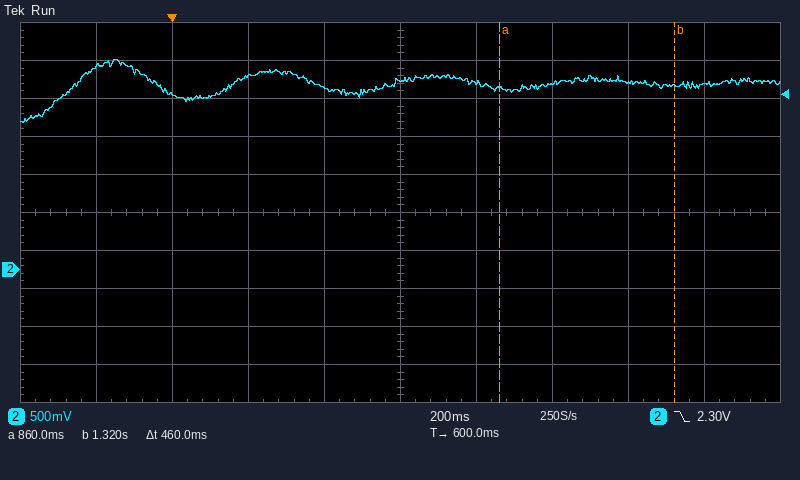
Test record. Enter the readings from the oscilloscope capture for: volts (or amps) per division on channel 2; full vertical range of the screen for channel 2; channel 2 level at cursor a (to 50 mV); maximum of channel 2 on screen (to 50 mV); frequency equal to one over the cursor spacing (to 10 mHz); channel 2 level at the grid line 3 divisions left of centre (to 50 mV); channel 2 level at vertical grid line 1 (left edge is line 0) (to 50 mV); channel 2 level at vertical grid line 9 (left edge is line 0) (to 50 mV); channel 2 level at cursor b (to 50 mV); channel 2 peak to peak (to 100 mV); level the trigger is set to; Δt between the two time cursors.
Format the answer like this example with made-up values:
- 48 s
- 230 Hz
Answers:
- 500 mV
- 5 V
- 2.40 V
- 2.75 V
- 2.17 Hz
- 2.30 V
- 2.65 V
- 2.45 V
- 2.40 V
- 800 mV
- 2.30 V
- 460 ms
